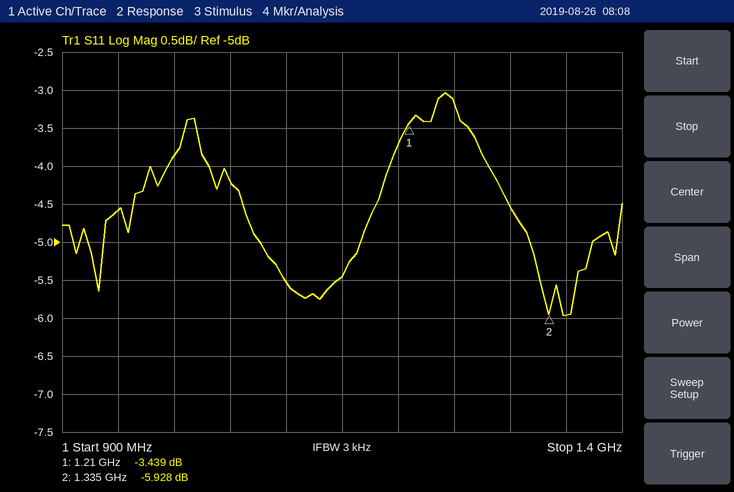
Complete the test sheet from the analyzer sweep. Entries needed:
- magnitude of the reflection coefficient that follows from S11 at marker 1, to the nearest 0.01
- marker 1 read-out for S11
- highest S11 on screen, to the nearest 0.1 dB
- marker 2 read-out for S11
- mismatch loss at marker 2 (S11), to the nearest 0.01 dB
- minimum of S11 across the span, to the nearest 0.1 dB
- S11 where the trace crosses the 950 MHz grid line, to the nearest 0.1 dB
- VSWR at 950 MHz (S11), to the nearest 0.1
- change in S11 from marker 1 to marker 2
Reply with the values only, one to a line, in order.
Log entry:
0.67
-3.439 dB
-3.0 dB
-5.928 dB
1.28 dB
-6.0 dB
-4.6 dB
3.9
-2.489 dB
